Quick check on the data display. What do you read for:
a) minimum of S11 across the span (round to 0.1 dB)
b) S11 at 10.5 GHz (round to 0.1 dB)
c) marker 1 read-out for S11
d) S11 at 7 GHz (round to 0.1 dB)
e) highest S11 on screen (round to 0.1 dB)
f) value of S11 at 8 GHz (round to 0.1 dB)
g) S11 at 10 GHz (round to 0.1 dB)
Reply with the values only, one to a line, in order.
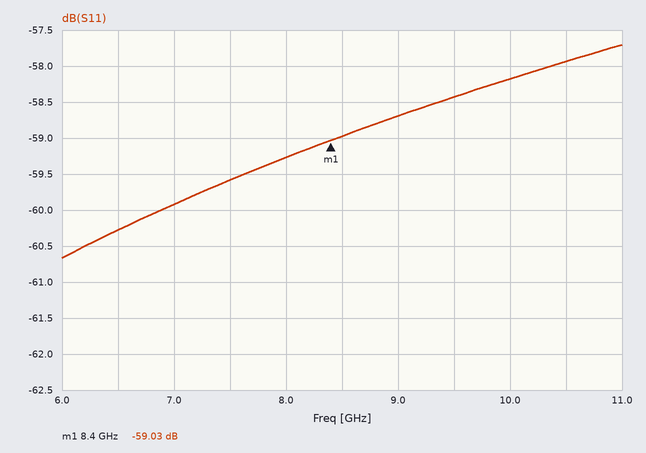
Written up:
-60.7 dB
-57.9 dB
-59.03 dB
-59.9 dB
-57.7 dB
-59.3 dB
-58.2 dB
